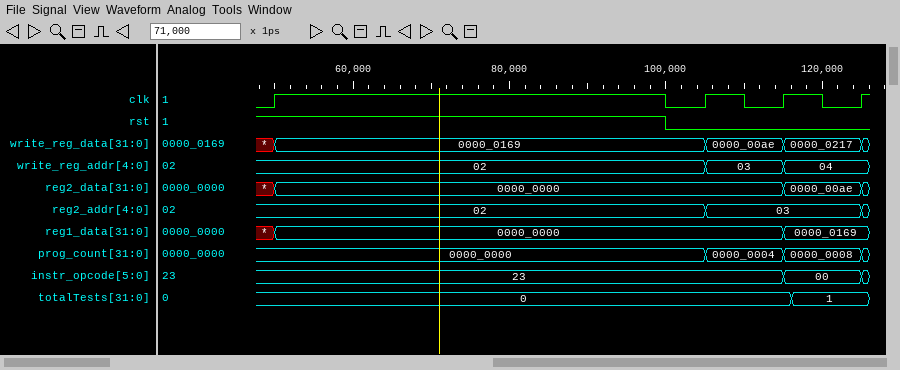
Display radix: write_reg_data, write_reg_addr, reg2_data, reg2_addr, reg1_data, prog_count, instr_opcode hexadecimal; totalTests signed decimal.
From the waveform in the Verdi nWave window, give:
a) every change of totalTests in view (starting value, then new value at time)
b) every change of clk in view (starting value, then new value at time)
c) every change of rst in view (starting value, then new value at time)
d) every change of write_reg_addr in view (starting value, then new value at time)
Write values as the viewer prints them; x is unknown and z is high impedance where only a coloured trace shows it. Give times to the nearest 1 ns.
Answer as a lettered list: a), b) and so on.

a) 0, 1 at 116 ns
b) 0, 1 at 50 ns, 0 at 100 ns, 1 at 105 ns, 0 at 110 ns, 1 at 115 ns, 0 at 120 ns, 1 at 125 ns
c) 1, 0 at 100 ns
d) 02, 03 at 105 ns, 04 at 115 ns
